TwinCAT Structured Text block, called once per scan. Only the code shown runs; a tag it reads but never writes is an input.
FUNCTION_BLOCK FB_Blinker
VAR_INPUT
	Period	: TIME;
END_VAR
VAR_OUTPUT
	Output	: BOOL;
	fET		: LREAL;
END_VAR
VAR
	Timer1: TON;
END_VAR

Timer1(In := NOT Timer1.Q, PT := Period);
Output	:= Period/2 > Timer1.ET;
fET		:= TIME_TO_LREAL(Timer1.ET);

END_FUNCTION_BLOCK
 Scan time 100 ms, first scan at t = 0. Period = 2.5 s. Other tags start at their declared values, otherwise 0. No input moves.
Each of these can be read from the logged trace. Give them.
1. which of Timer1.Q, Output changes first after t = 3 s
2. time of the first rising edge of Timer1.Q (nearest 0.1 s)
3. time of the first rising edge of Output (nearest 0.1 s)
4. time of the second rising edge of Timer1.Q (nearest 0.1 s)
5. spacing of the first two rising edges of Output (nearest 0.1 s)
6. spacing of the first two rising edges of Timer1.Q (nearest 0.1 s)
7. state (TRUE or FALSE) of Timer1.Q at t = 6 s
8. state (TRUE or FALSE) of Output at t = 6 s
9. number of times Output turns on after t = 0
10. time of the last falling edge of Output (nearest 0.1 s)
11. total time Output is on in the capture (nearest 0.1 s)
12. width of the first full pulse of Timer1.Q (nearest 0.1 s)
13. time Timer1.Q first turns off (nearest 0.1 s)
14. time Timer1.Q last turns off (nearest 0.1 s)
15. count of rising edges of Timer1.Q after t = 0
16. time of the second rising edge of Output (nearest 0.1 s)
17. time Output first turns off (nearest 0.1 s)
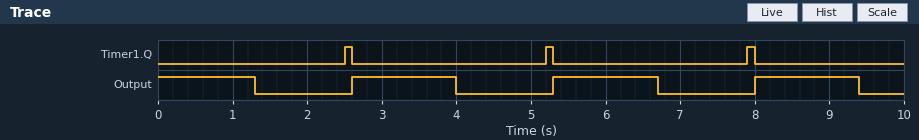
Output
2.5 s
2.6 s
5.2 s
2.7 s
2.7 s
FALSE
TRUE
3
9.4 s
5.5 s
0.1 s
2.6 s
8.0 s
3
5.3 s
1.3 s
